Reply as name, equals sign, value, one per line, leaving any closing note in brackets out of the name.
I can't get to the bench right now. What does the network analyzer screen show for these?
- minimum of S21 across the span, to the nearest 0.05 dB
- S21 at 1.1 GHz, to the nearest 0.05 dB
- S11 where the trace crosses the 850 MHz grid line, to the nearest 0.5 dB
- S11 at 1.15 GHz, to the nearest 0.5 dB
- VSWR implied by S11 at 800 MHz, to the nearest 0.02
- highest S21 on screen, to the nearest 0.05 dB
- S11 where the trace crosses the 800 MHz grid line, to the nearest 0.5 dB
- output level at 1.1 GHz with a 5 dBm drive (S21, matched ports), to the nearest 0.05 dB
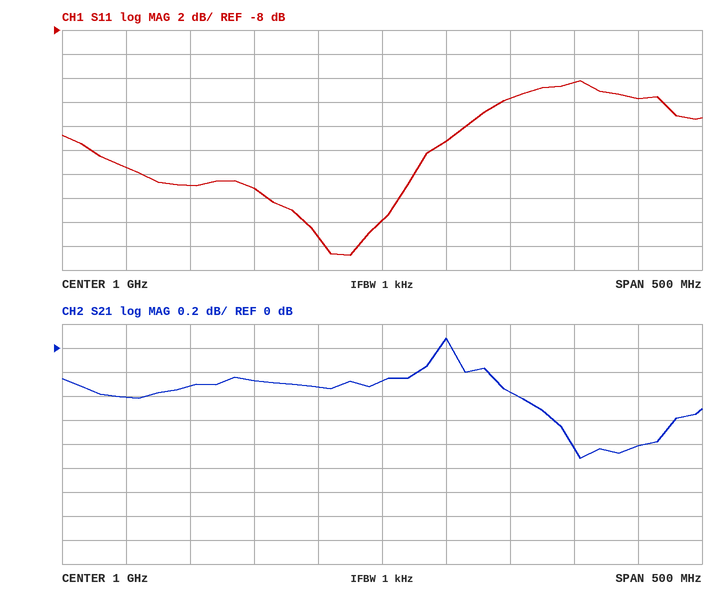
minimum of S21 across the span, to the nearest 0.05 dB = -0.90 dB
S21 at 1.1 GHz, to the nearest 0.05 dB = -0.35 dB
S11 where the trace crosses the 850 MHz grid line, to the nearest 0.5 dB = -21.0 dB
S11 at 1.15 GHz, to the nearest 0.5 dB = -12.5 dB
VSWR implied by S11 at 800 MHz, to the nearest 0.02 = 1.24
highest S21 on screen, to the nearest 0.05 dB = 0.10 dB
S11 where the trace crosses the 800 MHz grid line, to the nearest 0.5 dB = -19.5 dB
output level at 1.1 GHz with a 5 dBm drive (S21, matched ports), to the nearest 0.05 dB = 4.65 dBm
